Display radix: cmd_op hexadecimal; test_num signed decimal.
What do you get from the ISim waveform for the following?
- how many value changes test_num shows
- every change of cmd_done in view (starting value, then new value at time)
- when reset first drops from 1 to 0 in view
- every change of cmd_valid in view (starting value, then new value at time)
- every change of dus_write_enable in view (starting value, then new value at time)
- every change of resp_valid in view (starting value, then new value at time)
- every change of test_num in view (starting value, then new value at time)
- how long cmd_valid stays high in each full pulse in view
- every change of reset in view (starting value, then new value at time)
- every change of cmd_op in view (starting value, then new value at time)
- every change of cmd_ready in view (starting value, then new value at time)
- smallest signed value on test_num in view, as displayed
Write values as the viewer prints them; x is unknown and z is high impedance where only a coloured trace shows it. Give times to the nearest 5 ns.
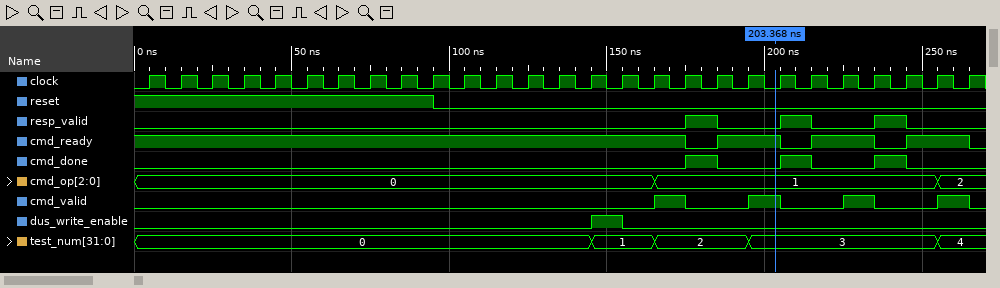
4
0, 1 at 175 ns, 0 at 185 ns, 1 at 205 ns, 0 at 215 ns, 1 at 235 ns, 0 at 245 ns
95 ns
0, 1 at 165 ns, 0 at 175 ns, 1 at 195 ns, 0 at 205 ns, 1 at 225 ns, 0 at 235 ns, 1 at 255 ns, 0 at 265 ns
0, 1 at 145 ns, 0 at 155 ns
0, 1 at 175 ns, 0 at 185 ns, 1 at 205 ns, 0 at 215 ns, 1 at 235 ns, 0 at 245 ns
0, 1 at 145 ns, 2 at 165 ns, 3 at 195 ns, 4 at 255 ns
10 ns, 10 ns, 10 ns, 10 ns
1, 0 at 95 ns
0, 1 at 165 ns, 2 at 255 ns
1, 0 at 175 ns, 1 at 185 ns, 0 at 205 ns, 1 at 215 ns, 0 at 235 ns, 1 at 245 ns, 0 at 265 ns
0
